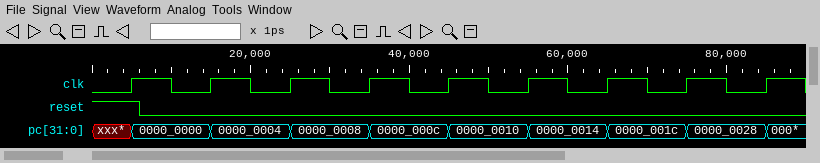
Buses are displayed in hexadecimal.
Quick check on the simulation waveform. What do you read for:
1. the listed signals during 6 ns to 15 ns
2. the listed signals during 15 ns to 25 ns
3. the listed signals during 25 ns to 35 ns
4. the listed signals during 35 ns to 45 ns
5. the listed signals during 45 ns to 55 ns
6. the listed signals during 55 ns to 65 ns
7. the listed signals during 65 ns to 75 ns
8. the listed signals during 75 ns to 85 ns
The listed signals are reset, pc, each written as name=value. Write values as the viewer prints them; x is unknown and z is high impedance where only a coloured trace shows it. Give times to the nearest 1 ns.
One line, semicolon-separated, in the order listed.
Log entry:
reset=0, pc=0000_0000; reset=0, pc=0000_0004; reset=0, pc=0000_0008; reset=0, pc=0000_000c; reset=0, pc=0000_0010; reset=0, pc=0000_0014; reset=0, pc=0000_001c; reset=0, pc=0000_0028
